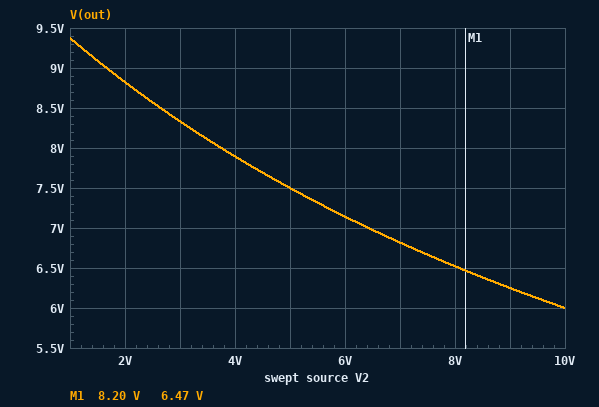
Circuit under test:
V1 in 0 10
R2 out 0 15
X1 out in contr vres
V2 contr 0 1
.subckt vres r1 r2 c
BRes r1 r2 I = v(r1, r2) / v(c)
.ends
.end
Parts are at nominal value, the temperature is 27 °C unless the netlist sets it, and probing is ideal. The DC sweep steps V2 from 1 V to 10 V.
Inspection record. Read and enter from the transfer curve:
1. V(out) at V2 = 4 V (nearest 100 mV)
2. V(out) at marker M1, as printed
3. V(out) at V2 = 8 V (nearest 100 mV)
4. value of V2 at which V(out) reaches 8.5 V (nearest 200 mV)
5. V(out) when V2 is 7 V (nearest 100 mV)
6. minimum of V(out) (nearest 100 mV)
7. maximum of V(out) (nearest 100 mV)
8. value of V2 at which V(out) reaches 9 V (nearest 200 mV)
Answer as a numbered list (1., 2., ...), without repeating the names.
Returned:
1. 7.9 V
2. 6.47 V
3. 6.5 V
4. 2.6 V
5. 6.8 V
6. 6.0 V
7. 9.4 V
8. 1.6 V
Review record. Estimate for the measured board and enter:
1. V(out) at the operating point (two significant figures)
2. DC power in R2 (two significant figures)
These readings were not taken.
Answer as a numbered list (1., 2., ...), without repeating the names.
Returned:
1. 9.4 V
2. 5.9 W
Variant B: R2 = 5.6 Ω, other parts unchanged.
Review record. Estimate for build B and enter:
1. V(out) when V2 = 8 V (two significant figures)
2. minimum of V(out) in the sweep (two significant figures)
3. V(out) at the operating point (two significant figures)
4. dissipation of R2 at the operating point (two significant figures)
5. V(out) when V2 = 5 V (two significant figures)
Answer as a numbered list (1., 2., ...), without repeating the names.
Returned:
1. 4.1 V
2. 3.6 V
3. 8.5 V
4. 13 W
5. 5.3 V
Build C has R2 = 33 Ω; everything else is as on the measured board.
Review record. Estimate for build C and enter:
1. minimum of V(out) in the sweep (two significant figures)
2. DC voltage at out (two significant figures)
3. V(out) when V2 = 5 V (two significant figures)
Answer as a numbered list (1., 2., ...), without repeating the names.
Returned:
1. 7.7 V
2. 9.7 V
3. 8.7 V
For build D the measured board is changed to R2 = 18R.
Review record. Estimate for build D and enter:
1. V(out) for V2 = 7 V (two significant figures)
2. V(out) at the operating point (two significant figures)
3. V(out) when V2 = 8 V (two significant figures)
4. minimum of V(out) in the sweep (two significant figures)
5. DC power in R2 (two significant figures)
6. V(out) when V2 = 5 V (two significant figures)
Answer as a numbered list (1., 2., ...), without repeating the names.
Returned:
1. 7.2 V
2. 9.5 V
3. 6.9 V
4. 6.4 V
5. 5.0 W
6. 7.8 V
